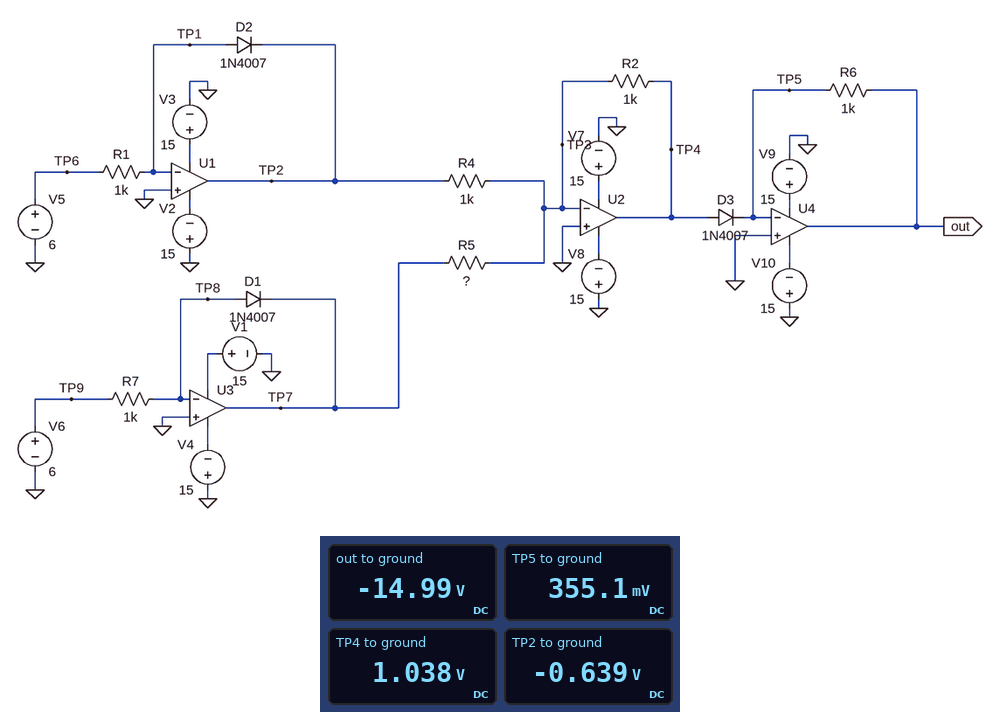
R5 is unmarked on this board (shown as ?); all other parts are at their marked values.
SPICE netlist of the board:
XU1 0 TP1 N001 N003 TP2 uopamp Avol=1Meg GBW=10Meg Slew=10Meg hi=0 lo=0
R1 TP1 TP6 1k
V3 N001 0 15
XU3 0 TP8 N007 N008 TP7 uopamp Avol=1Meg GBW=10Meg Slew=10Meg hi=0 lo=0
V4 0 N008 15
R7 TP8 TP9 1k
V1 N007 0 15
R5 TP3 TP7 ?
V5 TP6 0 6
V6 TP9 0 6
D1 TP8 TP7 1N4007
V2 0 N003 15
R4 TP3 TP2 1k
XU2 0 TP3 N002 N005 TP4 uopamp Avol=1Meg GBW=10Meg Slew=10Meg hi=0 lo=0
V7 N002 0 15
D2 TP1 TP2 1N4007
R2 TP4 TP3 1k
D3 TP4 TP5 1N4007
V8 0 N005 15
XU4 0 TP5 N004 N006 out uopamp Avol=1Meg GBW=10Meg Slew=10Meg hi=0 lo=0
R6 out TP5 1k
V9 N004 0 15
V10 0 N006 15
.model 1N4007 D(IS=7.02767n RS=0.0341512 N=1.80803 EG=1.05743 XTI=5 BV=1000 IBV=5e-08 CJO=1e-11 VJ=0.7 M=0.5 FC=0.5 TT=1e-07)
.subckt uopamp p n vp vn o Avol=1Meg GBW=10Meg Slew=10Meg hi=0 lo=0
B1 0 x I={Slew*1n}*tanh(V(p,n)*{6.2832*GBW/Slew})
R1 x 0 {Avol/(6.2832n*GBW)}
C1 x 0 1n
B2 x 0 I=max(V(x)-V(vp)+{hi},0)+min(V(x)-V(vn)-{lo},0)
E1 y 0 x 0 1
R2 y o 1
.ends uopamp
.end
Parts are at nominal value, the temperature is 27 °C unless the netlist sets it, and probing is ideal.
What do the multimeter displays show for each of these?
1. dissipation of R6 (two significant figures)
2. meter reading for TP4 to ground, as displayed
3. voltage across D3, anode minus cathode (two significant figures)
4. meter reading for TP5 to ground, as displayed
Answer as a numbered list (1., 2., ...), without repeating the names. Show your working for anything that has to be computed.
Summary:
1. (355.1 mV - (-14.99 V))^2 / 1 kΩ = 240 mW
2. 1.038 V
3. 1.038 V - 355.1 mV = 680 mV
4. 355.1 mV
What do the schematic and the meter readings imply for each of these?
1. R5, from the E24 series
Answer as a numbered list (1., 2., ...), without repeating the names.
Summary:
1. 1.6 kΩ
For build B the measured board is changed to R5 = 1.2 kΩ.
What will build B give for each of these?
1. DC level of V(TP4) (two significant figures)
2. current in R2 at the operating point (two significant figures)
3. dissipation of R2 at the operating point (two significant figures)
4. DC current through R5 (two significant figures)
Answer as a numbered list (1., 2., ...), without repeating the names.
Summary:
1. 1.2 V
2. 1.2 mA
3. 1.4 mW
4. 530 µA
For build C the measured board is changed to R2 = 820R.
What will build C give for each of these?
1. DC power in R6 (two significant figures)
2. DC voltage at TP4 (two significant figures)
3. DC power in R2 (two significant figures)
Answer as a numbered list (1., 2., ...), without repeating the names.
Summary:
1. 230 mW
2. 850 mV
3. 880 µW
